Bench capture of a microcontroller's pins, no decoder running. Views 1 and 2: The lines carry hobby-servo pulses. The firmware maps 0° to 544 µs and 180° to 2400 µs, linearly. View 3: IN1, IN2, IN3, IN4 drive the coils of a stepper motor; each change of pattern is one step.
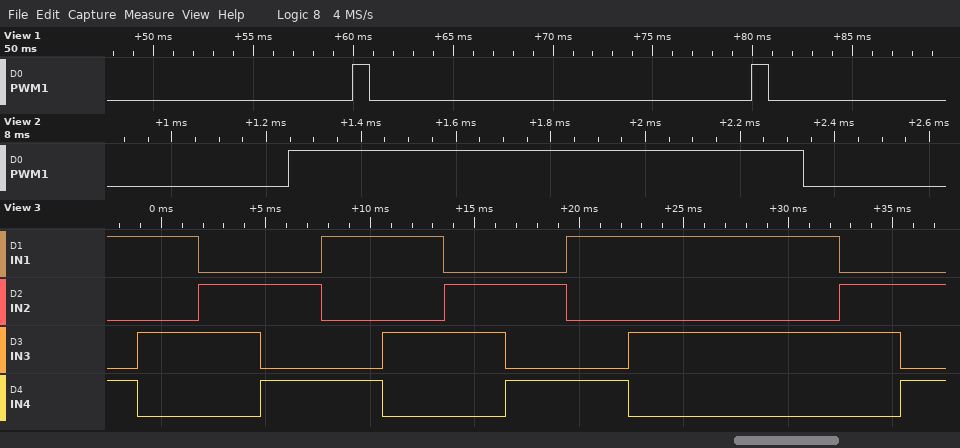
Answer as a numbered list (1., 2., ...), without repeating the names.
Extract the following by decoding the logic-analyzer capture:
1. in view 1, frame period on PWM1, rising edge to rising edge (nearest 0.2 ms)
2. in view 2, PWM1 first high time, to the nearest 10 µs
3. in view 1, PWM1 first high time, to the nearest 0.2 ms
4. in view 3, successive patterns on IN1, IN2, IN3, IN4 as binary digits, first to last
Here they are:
1. 20.0 ms
2. 1090 µs
3. 0.8 ms
4. 1001 1010 0110 0101 1001 1010 0110 0101 1001 1010 0110 0101
